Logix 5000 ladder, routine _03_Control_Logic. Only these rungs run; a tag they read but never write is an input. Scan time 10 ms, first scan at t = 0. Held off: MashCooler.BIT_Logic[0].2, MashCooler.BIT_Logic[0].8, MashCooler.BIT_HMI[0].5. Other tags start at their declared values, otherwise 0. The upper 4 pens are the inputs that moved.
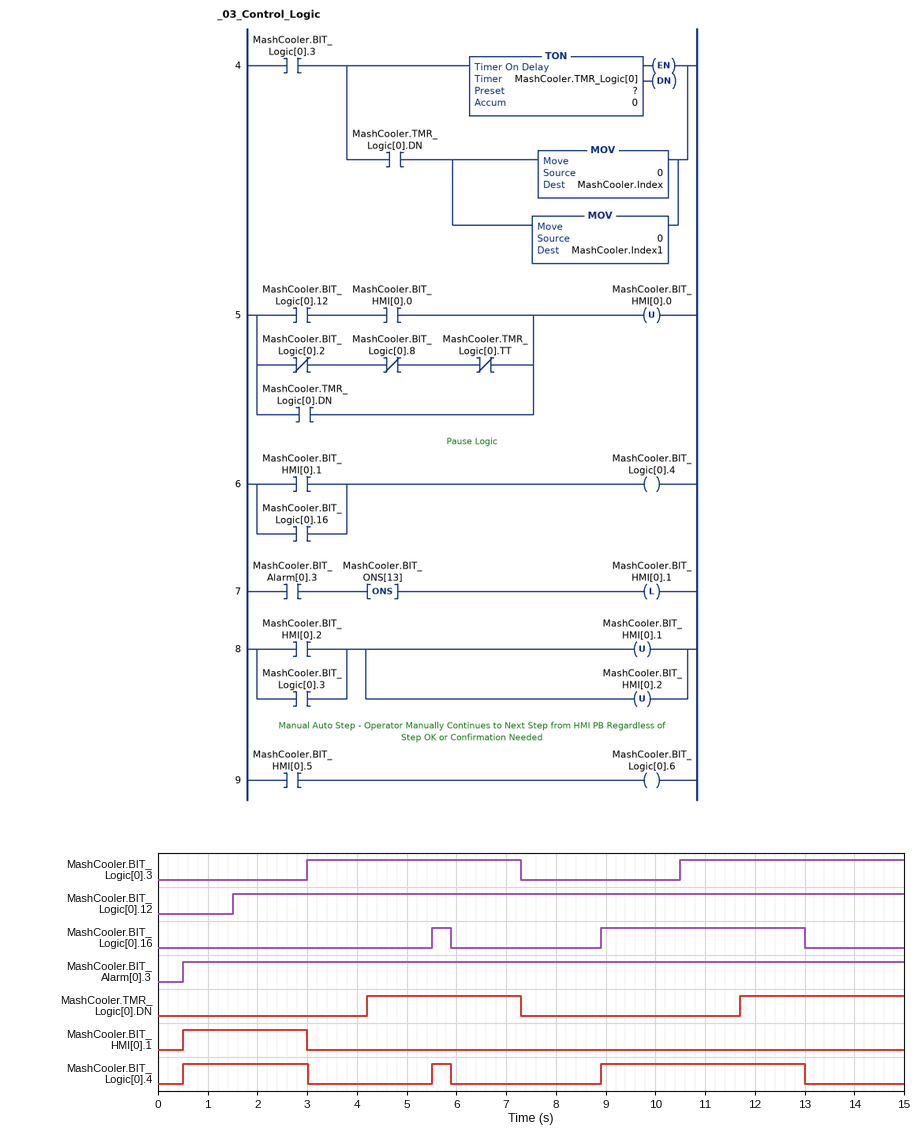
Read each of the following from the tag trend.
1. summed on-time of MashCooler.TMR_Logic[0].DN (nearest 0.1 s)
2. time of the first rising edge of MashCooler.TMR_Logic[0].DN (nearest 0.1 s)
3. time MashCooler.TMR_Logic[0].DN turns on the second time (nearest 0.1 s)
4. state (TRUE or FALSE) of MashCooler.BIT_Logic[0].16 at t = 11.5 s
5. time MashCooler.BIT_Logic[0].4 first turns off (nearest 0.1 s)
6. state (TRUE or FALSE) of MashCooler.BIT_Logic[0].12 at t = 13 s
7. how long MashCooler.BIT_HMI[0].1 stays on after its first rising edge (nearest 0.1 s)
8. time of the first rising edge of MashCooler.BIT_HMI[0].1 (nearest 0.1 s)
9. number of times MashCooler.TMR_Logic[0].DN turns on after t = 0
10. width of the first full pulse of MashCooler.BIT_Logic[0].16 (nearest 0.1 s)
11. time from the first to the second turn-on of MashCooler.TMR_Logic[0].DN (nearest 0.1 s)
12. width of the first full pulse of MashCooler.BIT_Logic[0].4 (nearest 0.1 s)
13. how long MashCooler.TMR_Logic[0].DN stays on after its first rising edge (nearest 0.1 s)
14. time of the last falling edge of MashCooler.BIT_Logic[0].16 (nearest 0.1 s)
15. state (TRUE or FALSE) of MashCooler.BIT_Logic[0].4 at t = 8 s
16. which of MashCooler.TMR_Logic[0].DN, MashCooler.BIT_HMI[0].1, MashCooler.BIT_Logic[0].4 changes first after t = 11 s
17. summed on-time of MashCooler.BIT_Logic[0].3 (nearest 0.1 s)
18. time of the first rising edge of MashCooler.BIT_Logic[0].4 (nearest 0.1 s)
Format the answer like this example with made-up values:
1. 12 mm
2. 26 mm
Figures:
1. 6.4 s
2. 4.2 s
3. 11.7 s
4. TRUE
5. 3.0 s
6. TRUE
7. 2.5 s
8. 0.5 s
9. 2
10. 0.4 s
11. 7.5 s
12. 2.5 s
13. 3.1 s
14. 13.0 s
15. FALSE
16. MashCooler.TMR_Logic[0].DN
17. 8.8 s
18. 0.5 s
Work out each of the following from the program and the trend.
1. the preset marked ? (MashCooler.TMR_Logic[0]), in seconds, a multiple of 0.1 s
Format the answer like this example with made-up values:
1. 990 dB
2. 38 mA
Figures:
1. 1.2 s
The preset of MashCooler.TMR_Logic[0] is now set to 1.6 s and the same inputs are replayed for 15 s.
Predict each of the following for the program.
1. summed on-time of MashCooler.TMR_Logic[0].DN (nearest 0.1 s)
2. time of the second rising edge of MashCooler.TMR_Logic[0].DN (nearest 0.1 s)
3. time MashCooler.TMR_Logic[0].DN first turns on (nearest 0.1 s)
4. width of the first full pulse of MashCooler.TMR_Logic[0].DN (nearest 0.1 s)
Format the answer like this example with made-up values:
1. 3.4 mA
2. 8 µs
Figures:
1. 5.6 s
2. 12.1 s
3. 4.6 s
4. 2.7 s
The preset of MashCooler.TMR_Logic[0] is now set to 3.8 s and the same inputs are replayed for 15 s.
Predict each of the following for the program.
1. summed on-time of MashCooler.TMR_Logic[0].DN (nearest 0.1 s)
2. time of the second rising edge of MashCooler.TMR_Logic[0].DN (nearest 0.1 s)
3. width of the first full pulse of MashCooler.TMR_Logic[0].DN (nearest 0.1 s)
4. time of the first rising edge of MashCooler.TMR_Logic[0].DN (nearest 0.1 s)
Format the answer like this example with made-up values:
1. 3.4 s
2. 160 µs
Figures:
1. 1.2 s
2. 14.3 s
3. 0.5 s
4. 6.8 s
